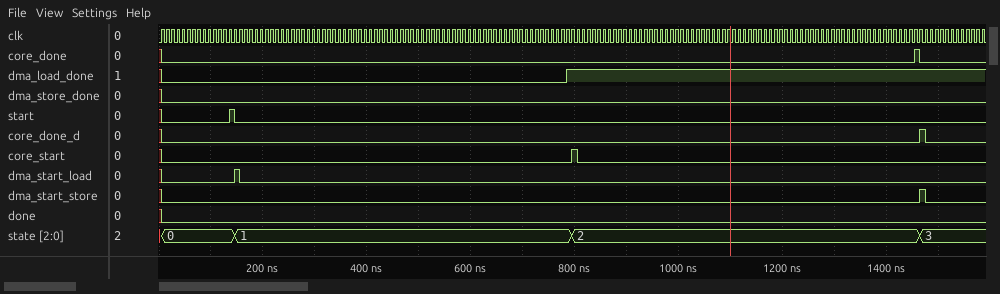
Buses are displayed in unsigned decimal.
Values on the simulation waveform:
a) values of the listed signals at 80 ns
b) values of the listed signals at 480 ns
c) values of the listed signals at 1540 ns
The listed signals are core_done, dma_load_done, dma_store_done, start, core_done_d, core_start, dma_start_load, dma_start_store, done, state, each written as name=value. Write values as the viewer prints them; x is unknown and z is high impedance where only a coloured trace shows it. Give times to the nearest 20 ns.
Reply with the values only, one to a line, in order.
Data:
core_done=0, dma_load_done=0, dma_store_done=0, start=0, core_done_d=0, core_start=0, dma_start_load=0, dma_start_store=0, done=0, state=0
core_done=0, dma_load_done=0, dma_store_done=0, start=0, core_done_d=0, core_start=0, dma_start_load=0, dma_start_store=0, done=0, state=1
core_done=0, dma_load_done=1, dma_store_done=0, start=0, core_done_d=0, core_start=0, dma_start_load=0, dma_start_store=0, done=0, state=3
